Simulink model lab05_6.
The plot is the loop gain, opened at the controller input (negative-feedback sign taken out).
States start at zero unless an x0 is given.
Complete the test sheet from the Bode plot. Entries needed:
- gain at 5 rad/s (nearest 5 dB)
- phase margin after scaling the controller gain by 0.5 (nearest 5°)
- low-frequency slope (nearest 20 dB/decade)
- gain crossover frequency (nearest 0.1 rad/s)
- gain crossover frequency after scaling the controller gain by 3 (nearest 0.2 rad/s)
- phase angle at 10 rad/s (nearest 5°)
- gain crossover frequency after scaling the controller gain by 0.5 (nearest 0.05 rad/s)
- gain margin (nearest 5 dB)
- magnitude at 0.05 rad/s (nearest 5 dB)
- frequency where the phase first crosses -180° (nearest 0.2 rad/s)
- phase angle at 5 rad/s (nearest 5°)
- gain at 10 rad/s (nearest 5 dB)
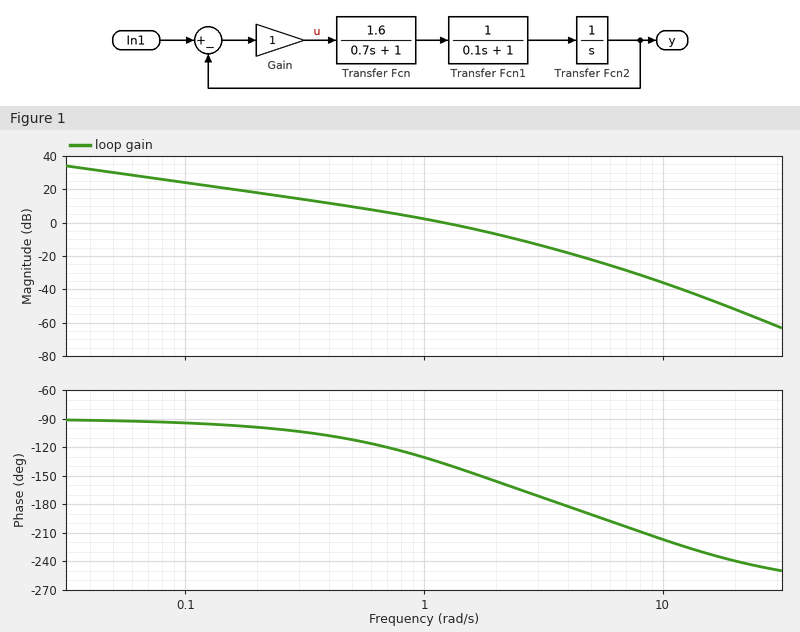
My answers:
-20 dB
60°
-20 dB/decade
1.2 rad/s
2.4 rad/s
-215°
0.70 rad/s
15 dB
30 dB
3.8 rad/s
-190°
-35 dB
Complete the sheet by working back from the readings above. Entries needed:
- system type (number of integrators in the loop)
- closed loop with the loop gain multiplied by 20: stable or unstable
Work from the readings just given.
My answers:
1
unstable
